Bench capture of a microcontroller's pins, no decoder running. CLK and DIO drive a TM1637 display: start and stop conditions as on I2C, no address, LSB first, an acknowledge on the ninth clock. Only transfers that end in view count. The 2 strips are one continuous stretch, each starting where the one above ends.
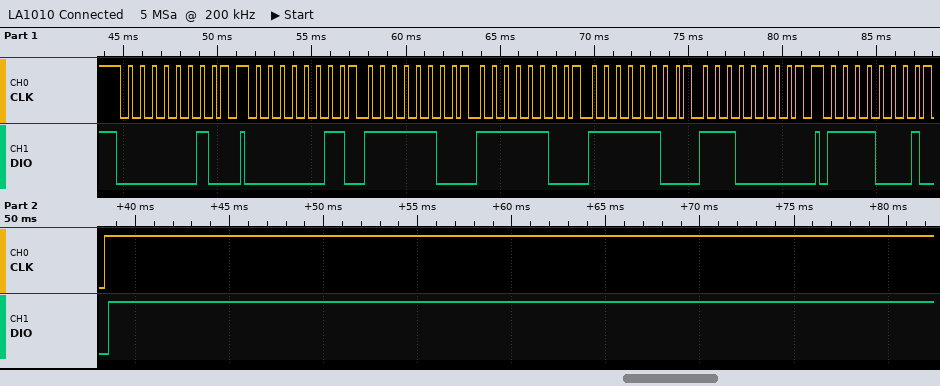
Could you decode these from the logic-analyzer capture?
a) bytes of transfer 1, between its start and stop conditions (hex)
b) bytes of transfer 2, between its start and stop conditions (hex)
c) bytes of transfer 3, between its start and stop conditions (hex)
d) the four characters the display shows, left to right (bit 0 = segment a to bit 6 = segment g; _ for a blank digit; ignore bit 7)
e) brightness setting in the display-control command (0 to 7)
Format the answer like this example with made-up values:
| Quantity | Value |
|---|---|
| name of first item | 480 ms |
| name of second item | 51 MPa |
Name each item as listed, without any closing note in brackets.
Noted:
| Quantity | Value |
|---|---|
| bytes of transfer 1, between its start and stop conditions | 40 |
| bytes of transfer 2, between its start and stop conditions | C0 3F 3F 3F 07 |
| bytes of transfer 3, between its start and stop conditions | 8F |
| the four characters the display shows, left to right | 0007 |
| brightness setting in the display-control command | 7 |
